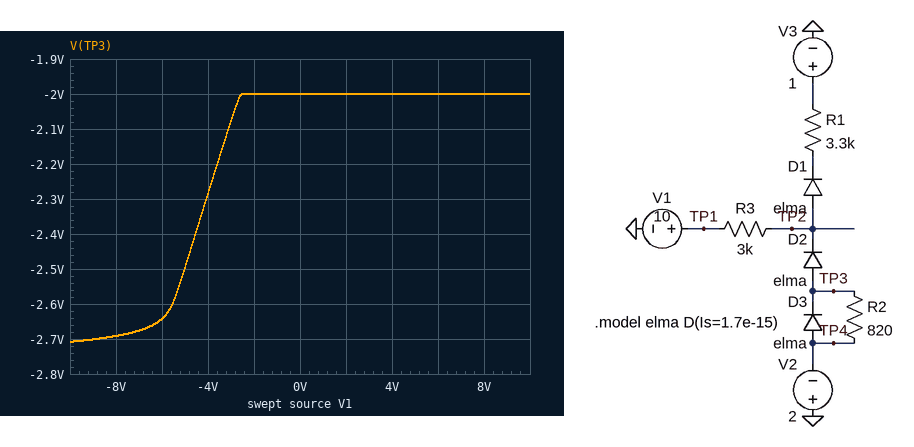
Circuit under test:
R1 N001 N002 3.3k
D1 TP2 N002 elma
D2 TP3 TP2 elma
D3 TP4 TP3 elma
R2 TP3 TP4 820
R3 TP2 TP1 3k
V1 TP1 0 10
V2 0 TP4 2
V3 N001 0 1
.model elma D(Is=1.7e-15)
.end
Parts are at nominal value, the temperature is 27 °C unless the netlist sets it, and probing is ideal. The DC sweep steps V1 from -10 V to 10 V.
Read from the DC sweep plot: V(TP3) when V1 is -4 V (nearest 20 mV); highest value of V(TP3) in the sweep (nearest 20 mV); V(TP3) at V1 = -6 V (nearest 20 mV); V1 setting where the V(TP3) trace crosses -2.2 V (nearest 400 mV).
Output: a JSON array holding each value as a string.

["-2.28 V", "-2.00 V", "-2.64 V", "-3.6 V"]
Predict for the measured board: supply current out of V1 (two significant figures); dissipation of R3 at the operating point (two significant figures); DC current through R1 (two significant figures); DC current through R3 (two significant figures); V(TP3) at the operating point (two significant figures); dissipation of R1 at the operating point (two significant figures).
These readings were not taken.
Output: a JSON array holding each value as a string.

["1.3 mA", "5.2 mW", "1.3 mA", "1.3 mA", "-2.0 V", "5.7 mW"]
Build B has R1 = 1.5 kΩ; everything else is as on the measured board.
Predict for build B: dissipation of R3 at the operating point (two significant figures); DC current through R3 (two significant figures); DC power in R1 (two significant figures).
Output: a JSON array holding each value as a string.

["10 mW", "1.8 mA", "5.1 mW"]
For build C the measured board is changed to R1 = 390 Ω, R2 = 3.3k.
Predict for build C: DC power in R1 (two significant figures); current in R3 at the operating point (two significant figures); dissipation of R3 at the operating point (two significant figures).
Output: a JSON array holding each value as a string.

["2.3 mW", "2.4 mA", "18 mW"]
